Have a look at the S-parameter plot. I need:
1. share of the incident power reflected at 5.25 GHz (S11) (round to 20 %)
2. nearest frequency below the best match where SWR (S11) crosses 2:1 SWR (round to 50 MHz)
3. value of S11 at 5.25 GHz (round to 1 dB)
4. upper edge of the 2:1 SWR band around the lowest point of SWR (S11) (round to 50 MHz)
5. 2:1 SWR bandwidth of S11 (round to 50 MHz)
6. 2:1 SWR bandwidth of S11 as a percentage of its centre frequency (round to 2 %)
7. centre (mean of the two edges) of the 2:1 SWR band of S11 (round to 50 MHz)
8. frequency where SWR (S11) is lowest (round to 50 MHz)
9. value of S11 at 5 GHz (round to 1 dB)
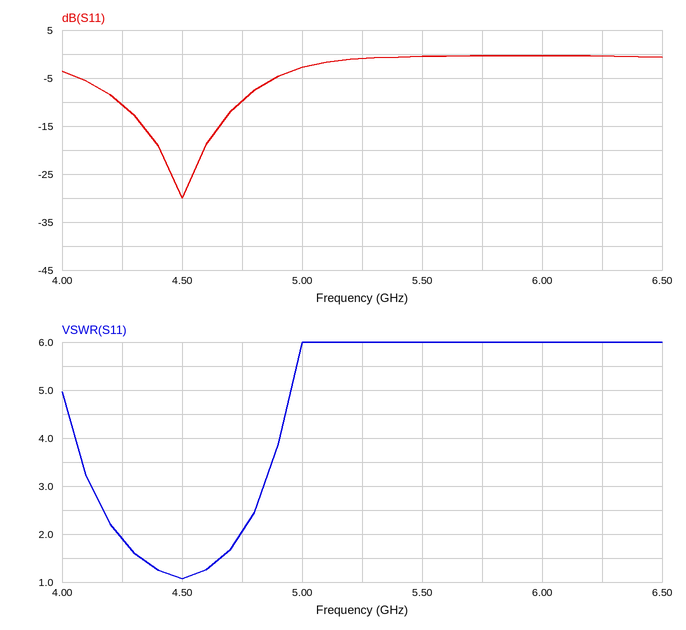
80 %
4.25 GHz
-1 dB
4.75 GHz
500 MHz
12 %
4.50 GHz
4.50 GHz
-3 dB
